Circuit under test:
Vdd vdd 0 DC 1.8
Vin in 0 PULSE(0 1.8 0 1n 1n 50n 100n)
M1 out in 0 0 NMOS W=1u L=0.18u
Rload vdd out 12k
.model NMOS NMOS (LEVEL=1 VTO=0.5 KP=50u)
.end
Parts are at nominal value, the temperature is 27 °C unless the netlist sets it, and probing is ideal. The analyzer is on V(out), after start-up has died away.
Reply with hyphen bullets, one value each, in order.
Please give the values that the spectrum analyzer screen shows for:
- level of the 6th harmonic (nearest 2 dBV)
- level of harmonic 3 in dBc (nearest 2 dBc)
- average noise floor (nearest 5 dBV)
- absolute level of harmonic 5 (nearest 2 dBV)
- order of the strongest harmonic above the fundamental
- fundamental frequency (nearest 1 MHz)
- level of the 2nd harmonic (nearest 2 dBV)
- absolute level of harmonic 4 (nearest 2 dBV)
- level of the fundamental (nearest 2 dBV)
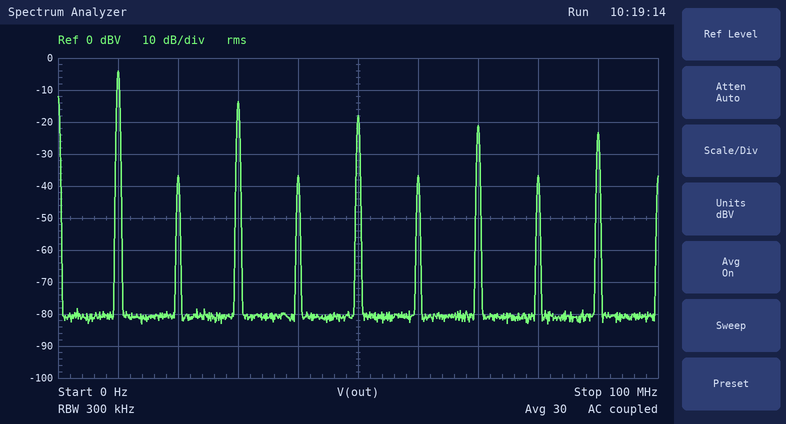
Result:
- -36 dBV
- -10 dBc
- -80 dBV
- -18 dBV
- 3
- 10 MHz
- -36 dBV
- -36 dBV
- -4 dBV
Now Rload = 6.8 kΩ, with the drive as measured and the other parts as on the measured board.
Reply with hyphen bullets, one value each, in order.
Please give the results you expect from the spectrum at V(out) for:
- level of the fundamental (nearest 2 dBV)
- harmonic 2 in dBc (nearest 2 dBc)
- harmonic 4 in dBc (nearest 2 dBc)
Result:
- -6 dBV
- -34 dBc
- -34 dBc
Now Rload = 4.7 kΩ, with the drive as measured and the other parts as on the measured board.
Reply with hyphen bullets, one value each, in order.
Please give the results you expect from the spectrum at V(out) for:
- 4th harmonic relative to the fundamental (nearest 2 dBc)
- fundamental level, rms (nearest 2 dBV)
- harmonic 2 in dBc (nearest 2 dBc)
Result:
- -36 dBc
- -8 dBV
- -36 dBc
